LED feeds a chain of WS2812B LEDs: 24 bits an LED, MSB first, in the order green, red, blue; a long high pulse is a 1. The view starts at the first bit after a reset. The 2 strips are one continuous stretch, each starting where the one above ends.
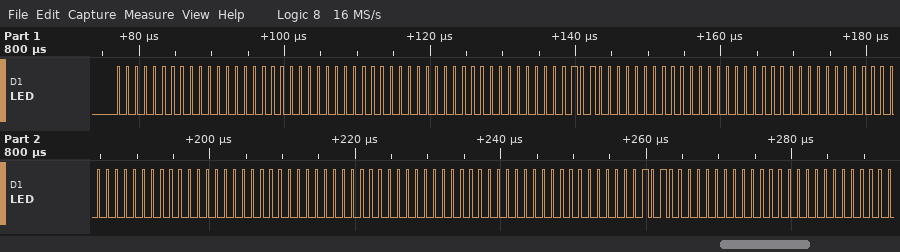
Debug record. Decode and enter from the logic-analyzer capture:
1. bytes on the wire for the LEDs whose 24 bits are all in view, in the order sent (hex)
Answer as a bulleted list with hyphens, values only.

- 00 00 00 00 00 00 28 00 00 00 00 00 00 00 00 00 00 00 28 00 00
